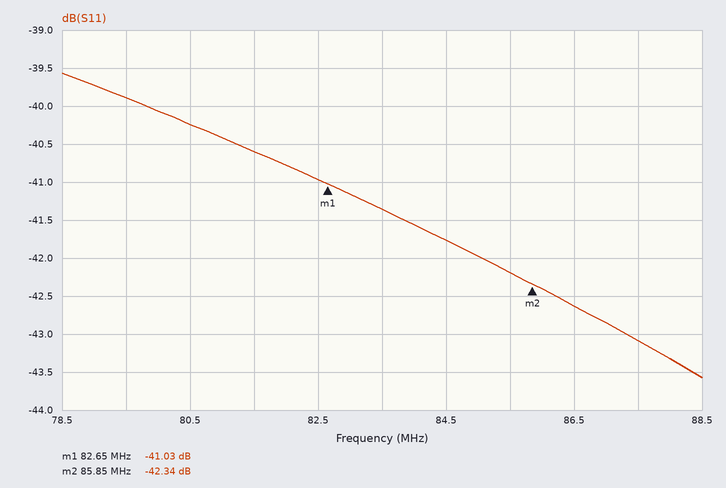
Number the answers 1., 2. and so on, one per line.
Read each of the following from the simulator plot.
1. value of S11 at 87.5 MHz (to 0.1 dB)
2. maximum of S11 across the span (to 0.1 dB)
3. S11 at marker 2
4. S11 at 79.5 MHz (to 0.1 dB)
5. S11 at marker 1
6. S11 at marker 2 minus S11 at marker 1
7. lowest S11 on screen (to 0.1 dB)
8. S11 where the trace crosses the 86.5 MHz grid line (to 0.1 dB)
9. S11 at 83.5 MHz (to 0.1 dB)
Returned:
1. -43.1 dB
2. -39.6 dB
3. -42.34 dB
4. -39.9 dB
5. -41.03 dB
6. -1.31 dB
7. -43.6 dB
8. -42.6 dB
9. -41.4 dB
